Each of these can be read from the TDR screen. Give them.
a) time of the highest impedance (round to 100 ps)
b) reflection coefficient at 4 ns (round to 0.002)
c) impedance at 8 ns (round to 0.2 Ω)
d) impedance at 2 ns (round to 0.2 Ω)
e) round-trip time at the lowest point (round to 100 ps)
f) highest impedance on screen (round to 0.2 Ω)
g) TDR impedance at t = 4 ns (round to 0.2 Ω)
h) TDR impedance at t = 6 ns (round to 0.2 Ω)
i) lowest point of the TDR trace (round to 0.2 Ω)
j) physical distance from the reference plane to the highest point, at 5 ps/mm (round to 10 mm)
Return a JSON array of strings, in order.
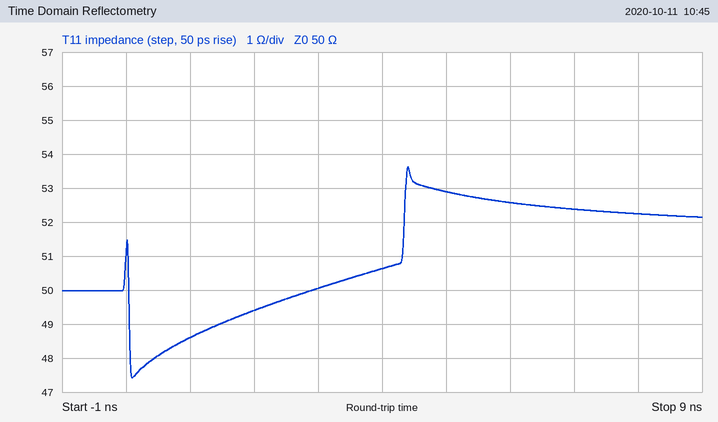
["4.4 ns", "+0.006", "52.2 Ω", "49.4 Ω", "100 ps", "53.6 Ω", "50.6 Ω", "52.6 Ω", "47.4 Ω", "440 mm"]
